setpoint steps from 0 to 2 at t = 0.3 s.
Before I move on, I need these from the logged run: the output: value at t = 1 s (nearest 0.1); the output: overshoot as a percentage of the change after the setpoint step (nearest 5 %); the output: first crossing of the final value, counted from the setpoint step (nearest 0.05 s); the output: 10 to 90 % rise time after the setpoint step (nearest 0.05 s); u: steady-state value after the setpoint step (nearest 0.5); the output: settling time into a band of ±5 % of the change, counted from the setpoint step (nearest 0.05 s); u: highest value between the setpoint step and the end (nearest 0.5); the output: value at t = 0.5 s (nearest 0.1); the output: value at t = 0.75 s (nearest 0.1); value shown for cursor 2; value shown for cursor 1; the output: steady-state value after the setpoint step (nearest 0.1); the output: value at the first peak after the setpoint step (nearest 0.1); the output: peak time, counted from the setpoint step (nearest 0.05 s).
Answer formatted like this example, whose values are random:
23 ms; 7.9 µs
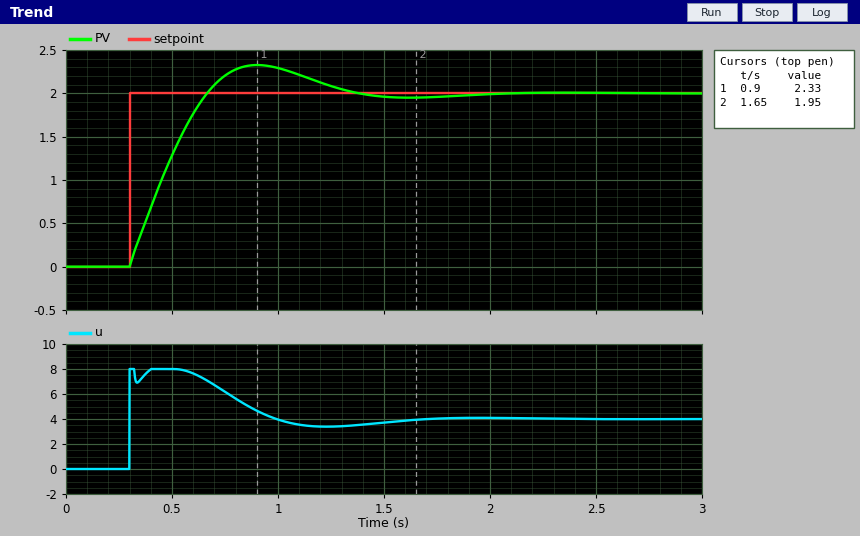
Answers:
2.3; 15 %; 0.35 s; 0.30 s; 4.0; 0.95 s; 8.0; 1.3; 2.2; 1.95; 2.33; 2.0; 2.3; 0.60 s
